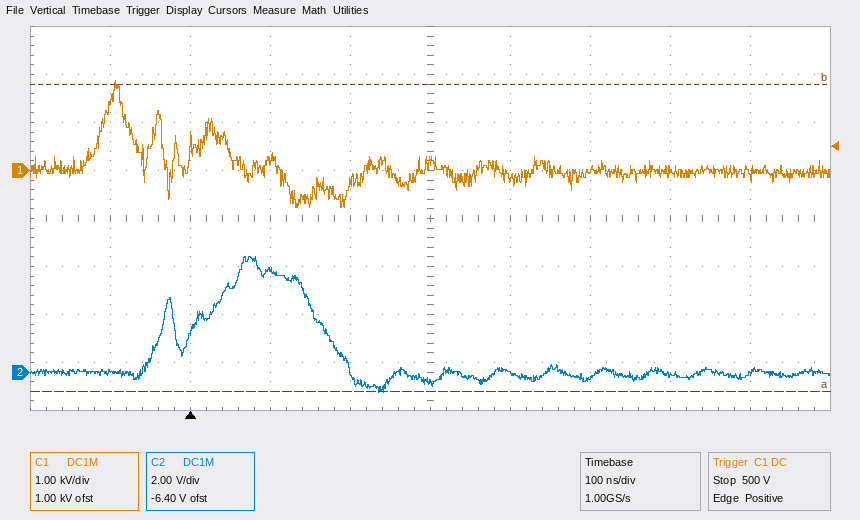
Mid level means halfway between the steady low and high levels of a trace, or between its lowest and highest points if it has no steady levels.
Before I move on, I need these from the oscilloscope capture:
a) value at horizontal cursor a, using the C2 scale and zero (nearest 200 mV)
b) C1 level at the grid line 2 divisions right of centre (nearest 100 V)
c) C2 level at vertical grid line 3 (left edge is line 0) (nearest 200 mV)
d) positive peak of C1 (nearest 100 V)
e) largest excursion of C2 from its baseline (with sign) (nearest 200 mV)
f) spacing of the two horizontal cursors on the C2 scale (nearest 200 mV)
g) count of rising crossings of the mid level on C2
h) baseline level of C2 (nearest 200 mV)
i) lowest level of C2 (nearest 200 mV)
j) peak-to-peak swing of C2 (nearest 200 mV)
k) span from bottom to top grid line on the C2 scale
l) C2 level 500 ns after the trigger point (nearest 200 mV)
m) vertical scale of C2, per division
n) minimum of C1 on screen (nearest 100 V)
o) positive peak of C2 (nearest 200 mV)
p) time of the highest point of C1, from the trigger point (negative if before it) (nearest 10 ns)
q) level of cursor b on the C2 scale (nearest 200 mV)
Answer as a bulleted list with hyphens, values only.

- -800 mV
- 0.0 kV
- 4.2 V
- 1.9 kV
- +4.8 V
- 12.8 V
- 2
- 0.0 V
- -800 mV
- 5.6 V
- 16 V
- -200 mV
- 2 V
- -800 V
- 4.8 V
- -90 ns
- 12.0 V
